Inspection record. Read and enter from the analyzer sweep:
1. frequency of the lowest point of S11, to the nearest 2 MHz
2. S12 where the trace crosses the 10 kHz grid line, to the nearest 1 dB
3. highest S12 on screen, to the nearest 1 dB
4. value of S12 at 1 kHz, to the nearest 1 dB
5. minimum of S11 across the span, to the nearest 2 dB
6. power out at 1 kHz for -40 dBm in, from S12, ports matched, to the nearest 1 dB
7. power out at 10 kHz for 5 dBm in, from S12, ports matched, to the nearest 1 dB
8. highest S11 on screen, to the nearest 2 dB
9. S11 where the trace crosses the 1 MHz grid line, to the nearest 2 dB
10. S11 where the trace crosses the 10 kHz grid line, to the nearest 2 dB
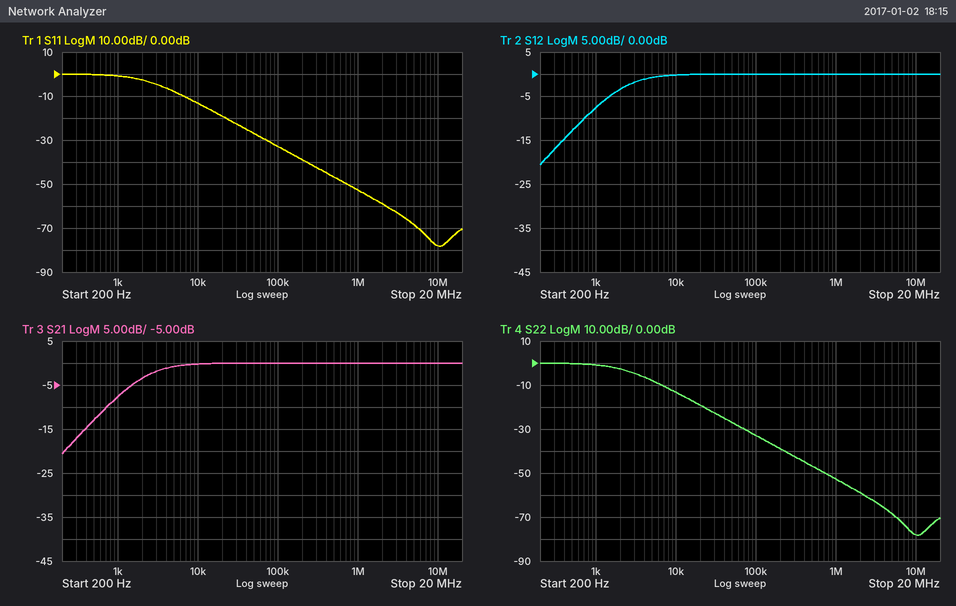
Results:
10 MHz
0 dB
0 dB
-8 dB
-78 dB
-48 dBm
5 dBm
0 dB
-52 dB
-14 dB
